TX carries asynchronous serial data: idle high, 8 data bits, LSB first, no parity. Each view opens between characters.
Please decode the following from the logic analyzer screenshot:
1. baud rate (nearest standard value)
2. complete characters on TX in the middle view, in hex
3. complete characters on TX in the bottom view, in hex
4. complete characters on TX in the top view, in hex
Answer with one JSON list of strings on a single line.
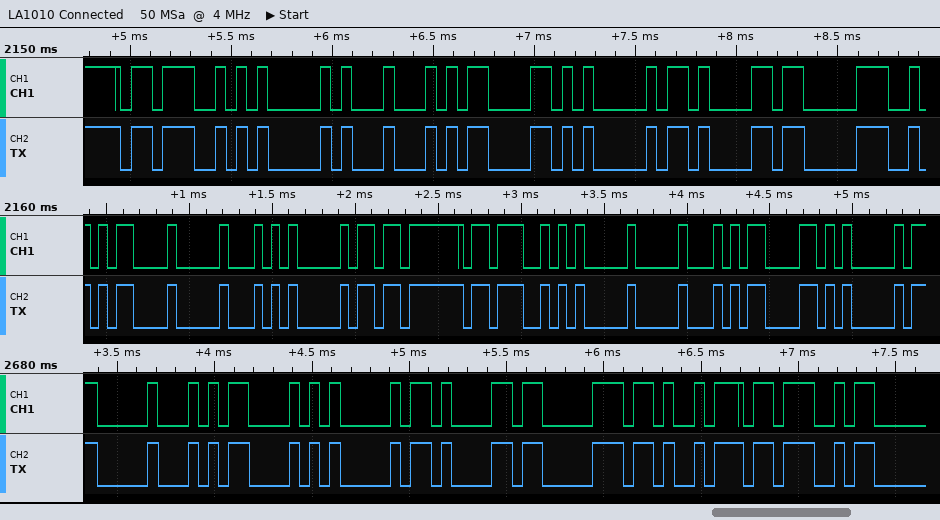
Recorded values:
["19200 baud", "0D, 10, 05, DB, 3B, 05, 10, 0D, 05", "10, 0D, 05, 0B, 83, 4B, 3B", "3B, 05, 11, 0D, 05, 0B, 83"]
